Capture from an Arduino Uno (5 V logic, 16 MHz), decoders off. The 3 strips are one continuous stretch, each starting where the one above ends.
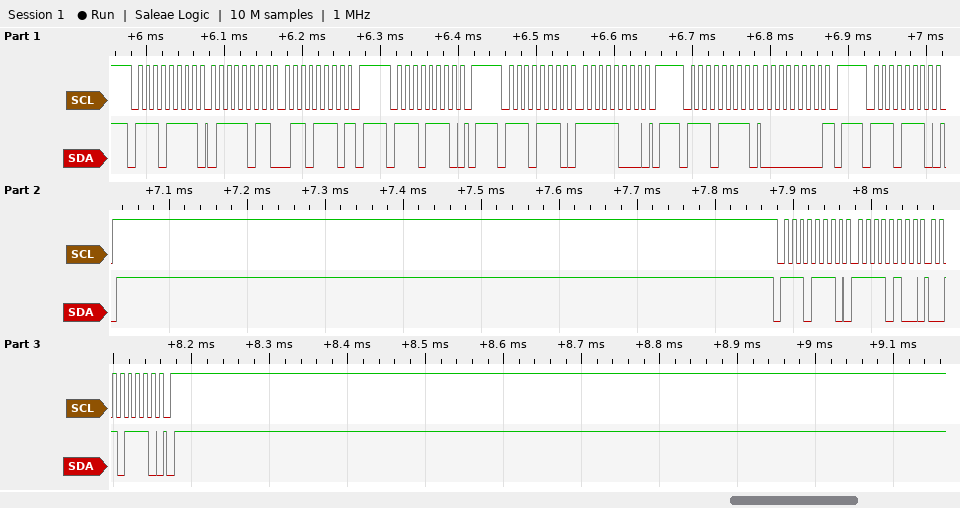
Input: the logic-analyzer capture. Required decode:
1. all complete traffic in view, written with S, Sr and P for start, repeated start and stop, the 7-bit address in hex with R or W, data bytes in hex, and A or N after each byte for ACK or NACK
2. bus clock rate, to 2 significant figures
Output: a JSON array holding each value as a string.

["S 77R A 7B A 6E N P S 77W A P S 77W A F8 A P S 77R A 00 N P S 77W A P S 77W A F4 A 2E A P", "100 kHz"]
